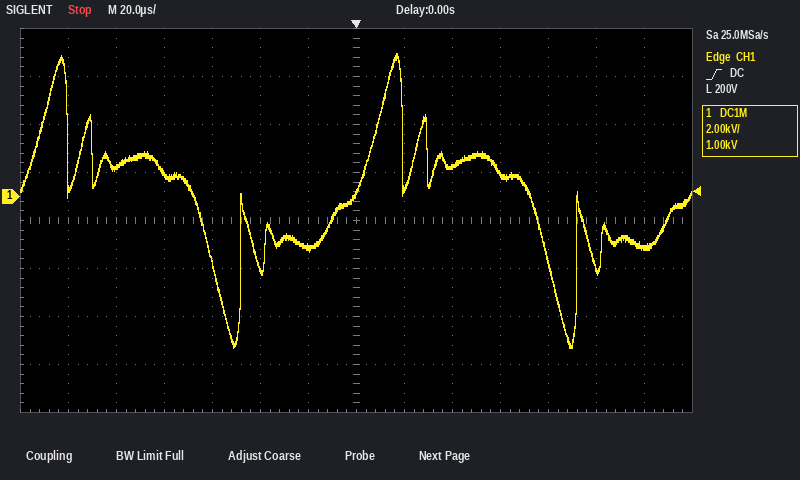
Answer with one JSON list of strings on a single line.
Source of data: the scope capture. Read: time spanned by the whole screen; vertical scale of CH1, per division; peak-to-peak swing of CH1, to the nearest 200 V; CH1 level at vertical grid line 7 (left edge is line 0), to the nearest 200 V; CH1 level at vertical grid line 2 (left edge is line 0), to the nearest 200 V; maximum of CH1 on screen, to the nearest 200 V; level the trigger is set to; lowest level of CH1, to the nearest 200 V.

["280 µs", "2 kV", "12.2 kV", "200 V", "1.2 kV", "6.0 kV", "200 V", "-6.2 kV"]
